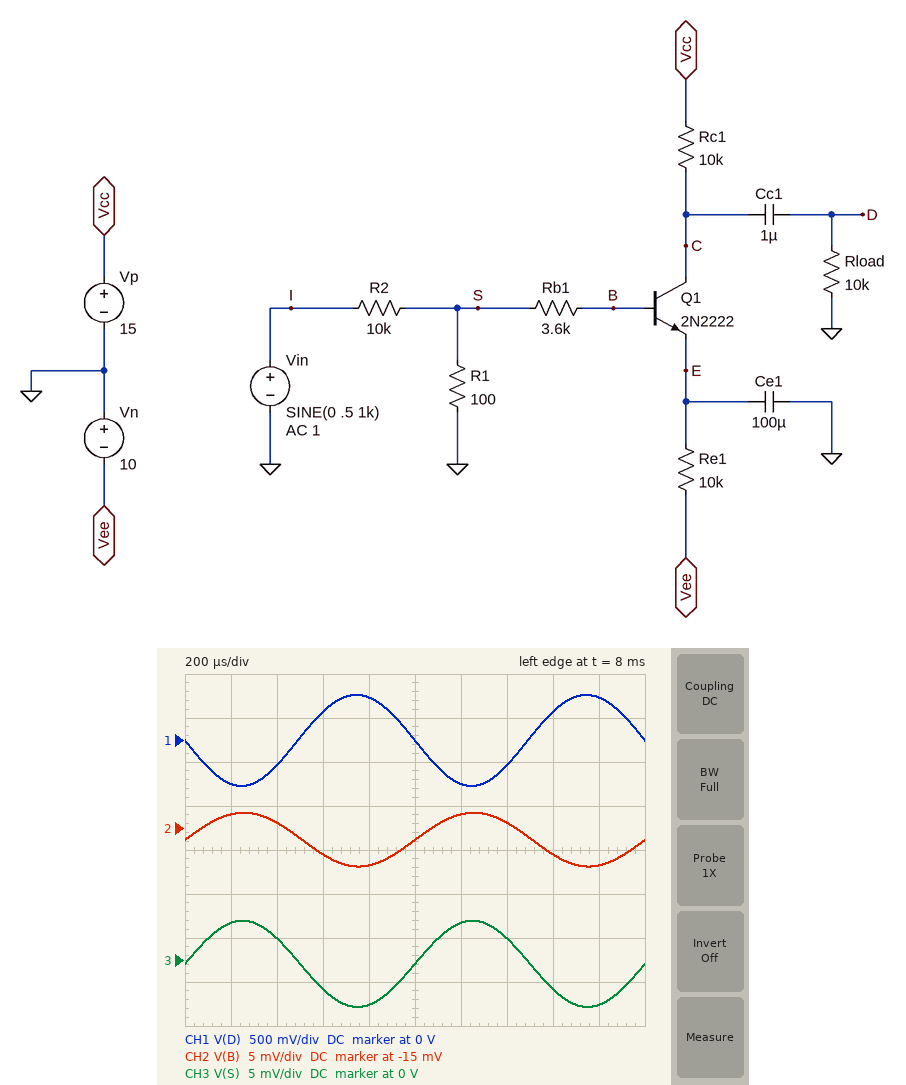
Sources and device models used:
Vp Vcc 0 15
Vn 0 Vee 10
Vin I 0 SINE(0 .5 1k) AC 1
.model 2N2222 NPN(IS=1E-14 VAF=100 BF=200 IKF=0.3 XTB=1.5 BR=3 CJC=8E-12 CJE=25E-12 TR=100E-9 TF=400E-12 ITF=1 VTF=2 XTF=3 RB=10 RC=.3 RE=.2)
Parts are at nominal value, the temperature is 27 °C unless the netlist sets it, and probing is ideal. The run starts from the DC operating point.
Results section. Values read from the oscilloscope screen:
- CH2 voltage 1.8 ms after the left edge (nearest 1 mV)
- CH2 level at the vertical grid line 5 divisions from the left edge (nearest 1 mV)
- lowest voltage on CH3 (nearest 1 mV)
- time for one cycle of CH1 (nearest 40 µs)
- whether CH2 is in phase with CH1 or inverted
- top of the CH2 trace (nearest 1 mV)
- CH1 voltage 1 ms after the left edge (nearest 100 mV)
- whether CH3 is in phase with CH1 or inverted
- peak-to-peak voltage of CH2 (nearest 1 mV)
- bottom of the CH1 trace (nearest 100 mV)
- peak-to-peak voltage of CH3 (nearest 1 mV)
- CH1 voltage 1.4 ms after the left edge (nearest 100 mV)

-19 mV
-16 mV
-5 mV
1.00 ms
inverted
-13 mV
0 V
inverted
6 mV
-500 mV
10 mV
-300 mV
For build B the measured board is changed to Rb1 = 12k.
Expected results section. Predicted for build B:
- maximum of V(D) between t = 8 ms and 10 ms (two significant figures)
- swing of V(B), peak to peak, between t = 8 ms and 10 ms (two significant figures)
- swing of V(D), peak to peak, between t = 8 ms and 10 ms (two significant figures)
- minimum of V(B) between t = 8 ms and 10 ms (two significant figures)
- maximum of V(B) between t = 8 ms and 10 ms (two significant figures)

280 mV
3.3 mV
550 mV
-55 mV
-51 mV
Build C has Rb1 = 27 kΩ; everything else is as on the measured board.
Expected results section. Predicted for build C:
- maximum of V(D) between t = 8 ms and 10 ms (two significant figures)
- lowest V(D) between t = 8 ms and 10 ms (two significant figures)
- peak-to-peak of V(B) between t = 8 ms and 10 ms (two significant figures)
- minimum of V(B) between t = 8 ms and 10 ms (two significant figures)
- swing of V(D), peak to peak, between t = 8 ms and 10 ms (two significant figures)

150 mV
-150 mV
1.8 mV
-120 mV
300 mV
